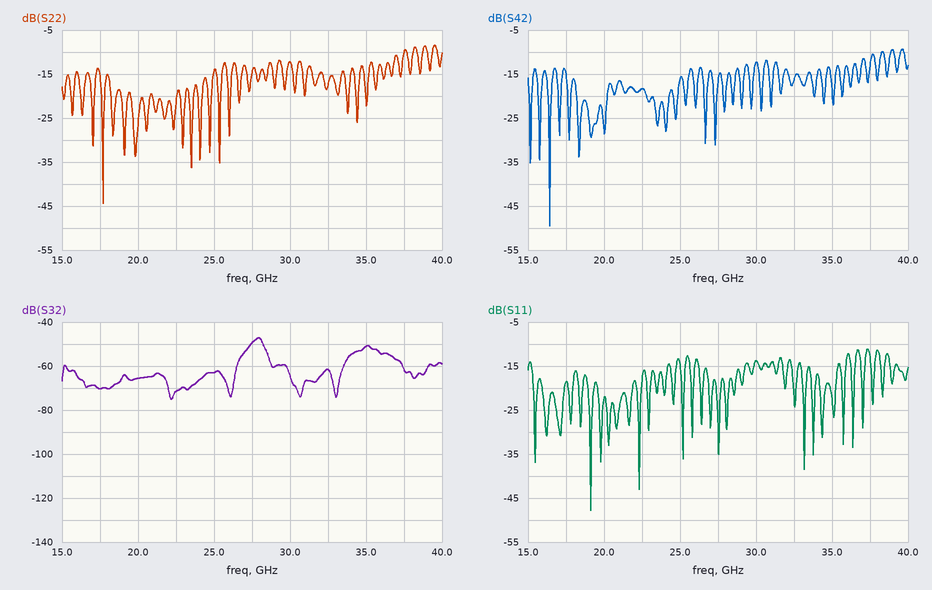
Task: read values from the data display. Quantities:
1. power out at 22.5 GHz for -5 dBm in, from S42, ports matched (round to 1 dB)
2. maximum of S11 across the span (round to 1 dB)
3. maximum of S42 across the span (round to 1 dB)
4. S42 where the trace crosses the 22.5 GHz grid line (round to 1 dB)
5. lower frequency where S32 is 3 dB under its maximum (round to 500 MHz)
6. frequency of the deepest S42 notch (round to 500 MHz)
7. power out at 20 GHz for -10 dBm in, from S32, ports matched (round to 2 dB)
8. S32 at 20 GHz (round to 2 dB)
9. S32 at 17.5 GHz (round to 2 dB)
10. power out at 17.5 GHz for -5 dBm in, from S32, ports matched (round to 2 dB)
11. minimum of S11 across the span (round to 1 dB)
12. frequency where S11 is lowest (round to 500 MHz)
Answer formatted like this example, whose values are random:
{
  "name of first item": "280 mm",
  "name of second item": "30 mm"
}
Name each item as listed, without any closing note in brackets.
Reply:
{
  "power out at 22.5 GHz for -5 dBm in, from S42, ports matched": "-23 dBm",
  "maximum of S11 across the span": "-11 dB",
  "maximum of S42 across the span": "-9 dB",
  "S42 where the trace crosses the 22.5 GHz grid line": "-18 dB",
  "lower frequency where S32 is 3 dB under its maximum": "27.5 GHz",
  "frequency of the deepest S42 notch": "16.5 GHz",
  "power out at 20 GHz for -10 dBm in, from S32, ports matched": "-76 dBm",
  "S32 at 20 GHz": "-66 dB",
  "S32 at 17.5 GHz": "-70 dB",
  "power out at 17.5 GHz for -5 dBm in, from S32, ports matched": "-76 dBm",
  "minimum of S11 across the span": "-48 dB",
  "frequency where S11 is lowest": "19.0 GHz"
}
